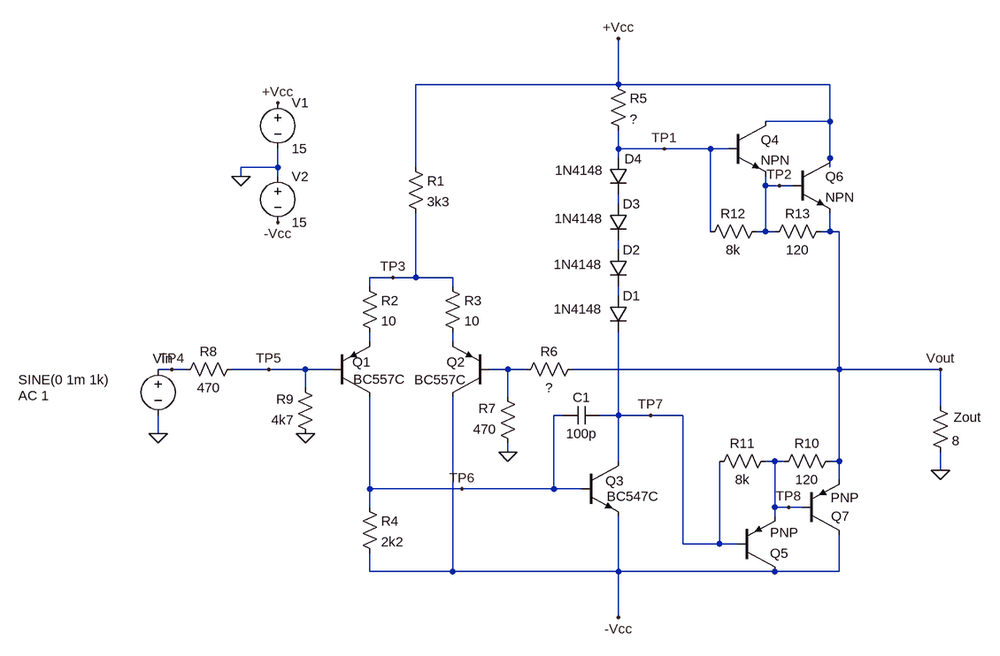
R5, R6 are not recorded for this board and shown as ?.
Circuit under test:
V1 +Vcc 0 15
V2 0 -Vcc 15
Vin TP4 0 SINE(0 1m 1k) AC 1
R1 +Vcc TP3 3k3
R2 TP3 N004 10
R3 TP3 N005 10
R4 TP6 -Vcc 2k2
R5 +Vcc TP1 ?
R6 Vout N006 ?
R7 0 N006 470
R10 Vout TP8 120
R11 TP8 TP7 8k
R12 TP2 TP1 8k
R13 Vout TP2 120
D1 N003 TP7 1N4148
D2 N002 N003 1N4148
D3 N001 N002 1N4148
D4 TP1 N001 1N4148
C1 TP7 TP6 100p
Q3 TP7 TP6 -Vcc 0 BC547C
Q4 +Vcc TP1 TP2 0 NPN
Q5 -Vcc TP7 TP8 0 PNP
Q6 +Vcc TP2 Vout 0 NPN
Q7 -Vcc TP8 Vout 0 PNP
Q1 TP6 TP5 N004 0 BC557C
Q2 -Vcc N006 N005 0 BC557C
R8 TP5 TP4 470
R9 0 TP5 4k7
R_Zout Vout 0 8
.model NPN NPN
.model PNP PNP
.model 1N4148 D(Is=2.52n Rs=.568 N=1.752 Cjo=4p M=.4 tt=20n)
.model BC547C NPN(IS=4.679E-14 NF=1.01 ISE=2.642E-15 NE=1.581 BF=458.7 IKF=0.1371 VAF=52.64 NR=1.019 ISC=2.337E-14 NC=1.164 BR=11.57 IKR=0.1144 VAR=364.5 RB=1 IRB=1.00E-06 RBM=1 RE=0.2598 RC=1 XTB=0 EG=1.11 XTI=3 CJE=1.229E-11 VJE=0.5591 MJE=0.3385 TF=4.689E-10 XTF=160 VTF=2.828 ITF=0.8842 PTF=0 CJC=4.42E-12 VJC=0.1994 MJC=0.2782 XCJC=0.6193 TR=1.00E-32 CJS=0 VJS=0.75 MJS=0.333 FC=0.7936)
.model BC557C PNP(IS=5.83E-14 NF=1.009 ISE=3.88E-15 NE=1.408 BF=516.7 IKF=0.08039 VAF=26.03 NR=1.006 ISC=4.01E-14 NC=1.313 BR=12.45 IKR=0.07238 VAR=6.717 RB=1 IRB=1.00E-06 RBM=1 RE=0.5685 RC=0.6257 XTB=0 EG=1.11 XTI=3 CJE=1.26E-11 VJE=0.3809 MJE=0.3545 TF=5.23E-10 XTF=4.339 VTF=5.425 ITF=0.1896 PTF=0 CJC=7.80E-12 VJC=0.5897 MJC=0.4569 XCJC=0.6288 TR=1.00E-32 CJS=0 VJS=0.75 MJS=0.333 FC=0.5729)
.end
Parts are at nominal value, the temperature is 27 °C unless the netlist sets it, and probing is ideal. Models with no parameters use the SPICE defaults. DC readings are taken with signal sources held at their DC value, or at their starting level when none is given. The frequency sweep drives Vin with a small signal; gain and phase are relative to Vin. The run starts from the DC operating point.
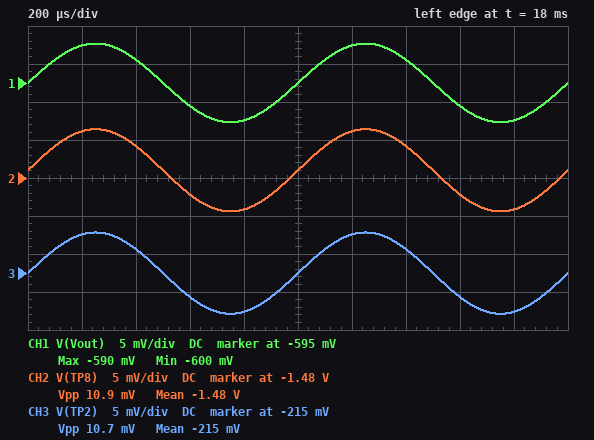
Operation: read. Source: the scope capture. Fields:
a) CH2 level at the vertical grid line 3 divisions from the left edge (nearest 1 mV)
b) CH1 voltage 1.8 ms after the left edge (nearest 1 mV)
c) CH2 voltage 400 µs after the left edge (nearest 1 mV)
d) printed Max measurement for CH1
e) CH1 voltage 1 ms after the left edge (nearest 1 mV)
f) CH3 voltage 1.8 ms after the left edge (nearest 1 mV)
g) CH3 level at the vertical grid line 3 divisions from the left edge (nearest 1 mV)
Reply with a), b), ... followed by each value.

a) -1.482 V
b) -600 mV
c) -1.476 V
d) -590 mV
e) -595 mV
f) -220 mV
g) -218 mV
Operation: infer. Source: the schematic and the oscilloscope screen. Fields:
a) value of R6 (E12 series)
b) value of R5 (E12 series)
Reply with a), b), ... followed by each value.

a) 2.2 kΩ
b) 820 Ω
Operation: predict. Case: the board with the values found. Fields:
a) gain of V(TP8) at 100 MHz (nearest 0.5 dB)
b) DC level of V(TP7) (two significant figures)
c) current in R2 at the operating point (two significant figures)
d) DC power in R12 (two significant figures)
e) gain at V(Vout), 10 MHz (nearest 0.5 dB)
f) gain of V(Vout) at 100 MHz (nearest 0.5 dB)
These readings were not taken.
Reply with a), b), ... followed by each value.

a) -35.5 dB
b) -2.3 V
c) 350 µA
d) 81 µW
e) 0.5 dB
f) -36.0 dB
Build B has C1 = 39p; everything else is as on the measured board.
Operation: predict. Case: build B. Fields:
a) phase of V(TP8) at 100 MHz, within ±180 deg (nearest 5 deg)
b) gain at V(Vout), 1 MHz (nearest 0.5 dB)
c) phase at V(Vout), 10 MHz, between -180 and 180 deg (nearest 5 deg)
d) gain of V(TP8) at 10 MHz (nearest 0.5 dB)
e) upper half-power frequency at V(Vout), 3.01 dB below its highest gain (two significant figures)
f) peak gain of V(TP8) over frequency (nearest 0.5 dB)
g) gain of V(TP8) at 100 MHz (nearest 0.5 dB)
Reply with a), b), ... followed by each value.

a) 150 deg
b) 14.5 dB
c) -115 deg
d) 10.5 dB
e) 8.8 MHz
f) 15.0 dB
g) -27.5 dB
